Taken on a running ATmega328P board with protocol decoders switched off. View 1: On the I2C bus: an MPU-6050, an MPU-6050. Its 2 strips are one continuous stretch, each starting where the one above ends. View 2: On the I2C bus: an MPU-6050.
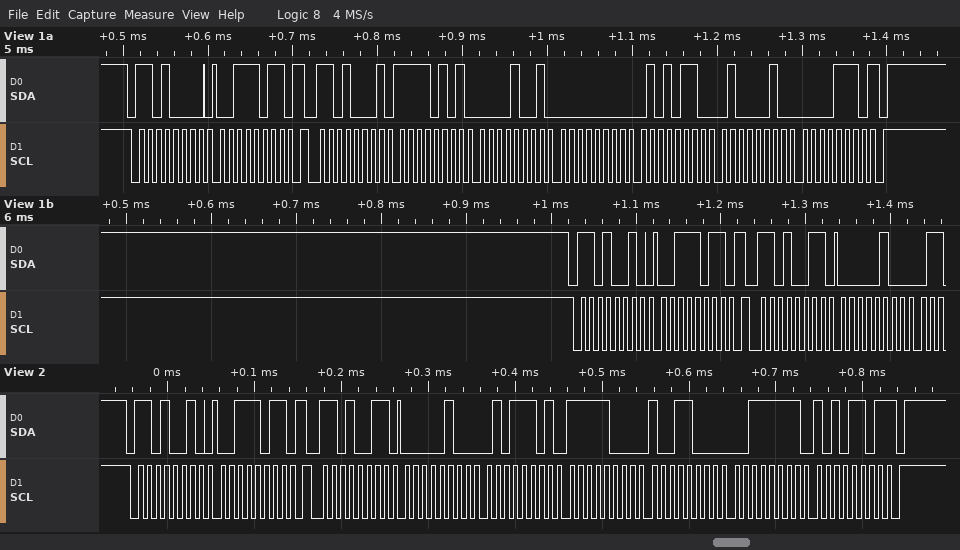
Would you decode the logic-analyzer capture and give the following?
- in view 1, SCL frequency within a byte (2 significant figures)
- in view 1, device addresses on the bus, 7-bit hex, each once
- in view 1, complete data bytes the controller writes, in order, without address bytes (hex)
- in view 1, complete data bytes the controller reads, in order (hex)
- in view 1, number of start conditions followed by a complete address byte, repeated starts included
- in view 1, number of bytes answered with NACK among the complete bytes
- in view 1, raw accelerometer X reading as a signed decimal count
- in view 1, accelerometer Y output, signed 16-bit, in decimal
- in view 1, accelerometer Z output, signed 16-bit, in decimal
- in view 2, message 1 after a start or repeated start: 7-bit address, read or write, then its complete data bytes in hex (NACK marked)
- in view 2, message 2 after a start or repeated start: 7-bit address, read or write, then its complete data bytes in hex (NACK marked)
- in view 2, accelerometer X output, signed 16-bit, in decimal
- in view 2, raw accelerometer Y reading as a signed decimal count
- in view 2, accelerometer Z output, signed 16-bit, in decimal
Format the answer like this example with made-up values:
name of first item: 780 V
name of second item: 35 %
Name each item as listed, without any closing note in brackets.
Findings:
in view 1, SCL frequency within a byte: 100 kHz
in view 1, device addresses on the bus, 7-bit hex, each once: 0x68 0x69
in view 1, complete data bytes the controller writes, in order, without address bytes: 3B 3B
in view 1, complete data bytes the controller reads, in order: F5 09 00 56 42 0E 04
in view 1, number of start conditions followed by a complete address byte, repeated starts included: 4
in view 1, number of bytes answered with NACK among the complete bytes: 1
in view 1, raw accelerometer X reading as a signed decimal count: -2807
in view 1, accelerometer Y output, signed 16-bit, in decimal: 86
in view 1, accelerometer Z output, signed 16-bit, in decimal: 16910
in view 2, message 1 after a start or repeated start: 7-bit address, read or write, then its complete data bytes in hex: 0x69 write: 3B
in view 2, message 2 after a start or repeated start: 7-bit address, read or write, then its complete data bytes in hex: 0x69 read: 04 5D F8 98 3F AD NACK
in view 2, accelerometer X output, signed 16-bit, in decimal: 1117
in view 2, raw accelerometer Y reading as a signed decimal count: -1896
in view 2, accelerometer Z output, signed 16-bit, in decimal: 16301
